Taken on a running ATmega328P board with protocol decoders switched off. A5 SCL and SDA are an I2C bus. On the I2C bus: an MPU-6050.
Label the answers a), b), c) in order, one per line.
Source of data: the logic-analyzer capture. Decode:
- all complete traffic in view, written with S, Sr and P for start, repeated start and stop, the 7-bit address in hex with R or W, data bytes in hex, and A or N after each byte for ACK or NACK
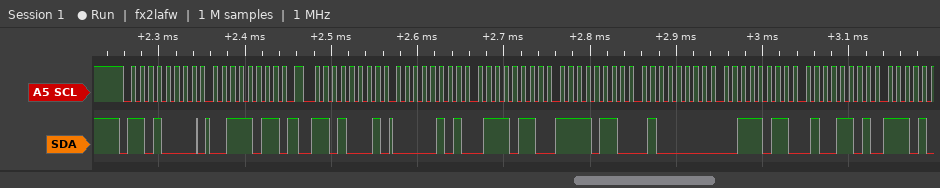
a) S 68W A 3B A Sr 68R A 05 A 76 A F6 A 40 A 3B A 4D A
